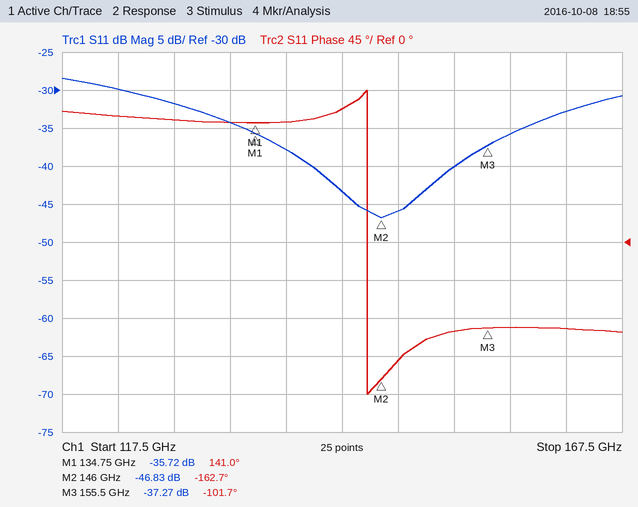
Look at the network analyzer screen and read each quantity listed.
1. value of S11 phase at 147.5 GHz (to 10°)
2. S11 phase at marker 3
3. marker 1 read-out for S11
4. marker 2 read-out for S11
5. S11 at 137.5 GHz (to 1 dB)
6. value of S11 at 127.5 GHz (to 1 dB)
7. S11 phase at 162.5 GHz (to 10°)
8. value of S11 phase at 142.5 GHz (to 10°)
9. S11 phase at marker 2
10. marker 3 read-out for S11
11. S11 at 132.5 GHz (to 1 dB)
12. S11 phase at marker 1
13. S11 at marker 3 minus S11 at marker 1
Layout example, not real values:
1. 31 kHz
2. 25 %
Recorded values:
1. -140°
2. -101.7°
3. -35.72 dB
4. -46.83 dB
5. -38 dB
6. -32 dB
7. -100°
8. 160°
9. -162.7°
10. -37.27 dB
11. -34 dB
12. 141.0°
13. -1.55 dB
